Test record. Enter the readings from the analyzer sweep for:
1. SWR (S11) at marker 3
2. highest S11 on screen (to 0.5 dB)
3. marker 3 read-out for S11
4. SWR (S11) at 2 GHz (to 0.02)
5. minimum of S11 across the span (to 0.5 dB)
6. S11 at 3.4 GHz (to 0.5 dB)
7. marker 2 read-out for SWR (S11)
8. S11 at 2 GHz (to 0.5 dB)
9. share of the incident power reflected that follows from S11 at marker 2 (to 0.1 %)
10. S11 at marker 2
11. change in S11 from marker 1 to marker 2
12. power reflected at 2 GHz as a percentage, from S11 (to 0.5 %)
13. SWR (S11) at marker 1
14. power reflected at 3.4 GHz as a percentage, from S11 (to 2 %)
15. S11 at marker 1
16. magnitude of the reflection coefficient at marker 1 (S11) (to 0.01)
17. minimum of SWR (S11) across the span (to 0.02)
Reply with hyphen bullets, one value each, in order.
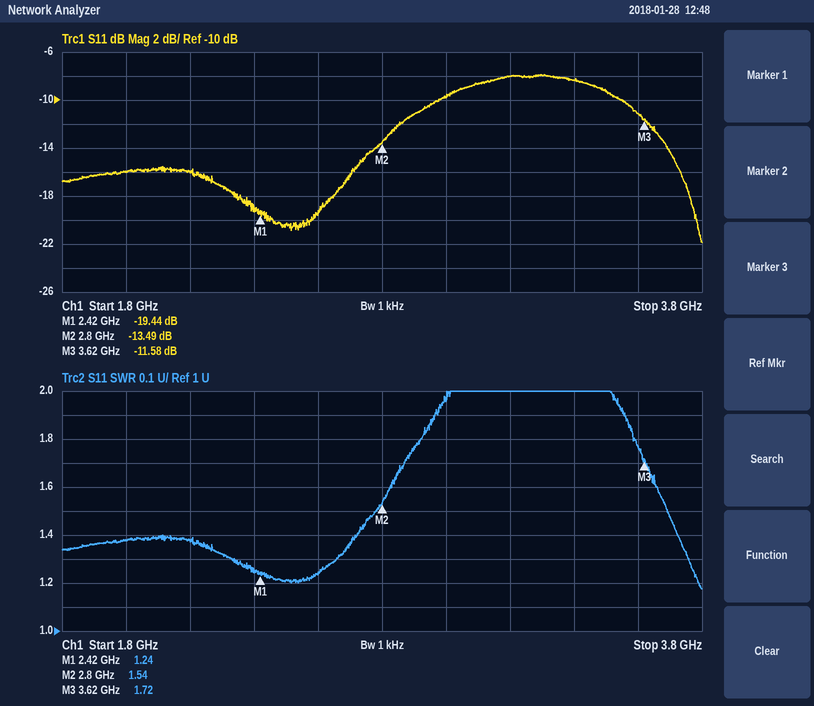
- 1.72
- -8.0 dB
- -11.58 dB
- 1.38
- -22.0 dB
- -8.5 dB
- 1.54
- -16.0 dB
- 4.5 %
- -13.49 dB
- 5.95 dB
- 2.5 %
- 1.24
- 14 %
- -19.44 dB
- 0.11
- 1.18
